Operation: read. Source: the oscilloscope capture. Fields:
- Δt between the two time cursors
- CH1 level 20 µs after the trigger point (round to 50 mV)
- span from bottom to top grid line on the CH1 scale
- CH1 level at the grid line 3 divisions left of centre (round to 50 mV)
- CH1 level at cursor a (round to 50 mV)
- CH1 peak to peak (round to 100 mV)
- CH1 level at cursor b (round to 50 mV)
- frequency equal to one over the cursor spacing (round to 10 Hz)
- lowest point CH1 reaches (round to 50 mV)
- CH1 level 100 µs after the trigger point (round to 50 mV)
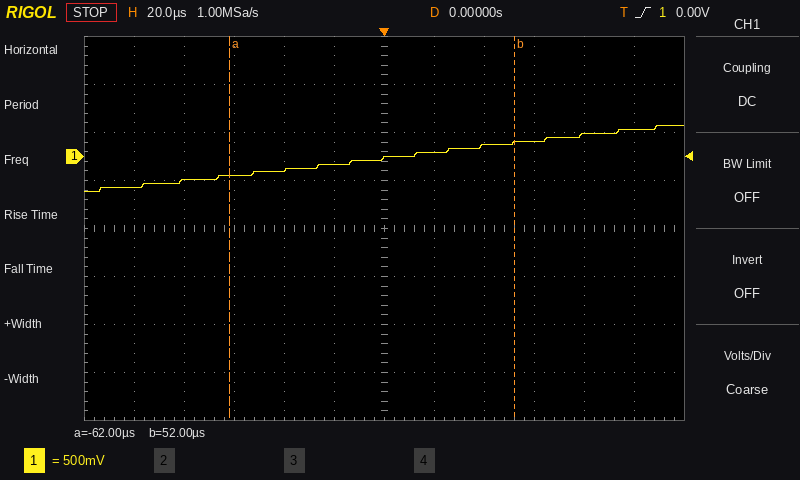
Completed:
114 µs
50 mV
4 V
-200 mV
-200 mV
700 mV
150 mV
8.77 kHz
-350 mV
300 mV
